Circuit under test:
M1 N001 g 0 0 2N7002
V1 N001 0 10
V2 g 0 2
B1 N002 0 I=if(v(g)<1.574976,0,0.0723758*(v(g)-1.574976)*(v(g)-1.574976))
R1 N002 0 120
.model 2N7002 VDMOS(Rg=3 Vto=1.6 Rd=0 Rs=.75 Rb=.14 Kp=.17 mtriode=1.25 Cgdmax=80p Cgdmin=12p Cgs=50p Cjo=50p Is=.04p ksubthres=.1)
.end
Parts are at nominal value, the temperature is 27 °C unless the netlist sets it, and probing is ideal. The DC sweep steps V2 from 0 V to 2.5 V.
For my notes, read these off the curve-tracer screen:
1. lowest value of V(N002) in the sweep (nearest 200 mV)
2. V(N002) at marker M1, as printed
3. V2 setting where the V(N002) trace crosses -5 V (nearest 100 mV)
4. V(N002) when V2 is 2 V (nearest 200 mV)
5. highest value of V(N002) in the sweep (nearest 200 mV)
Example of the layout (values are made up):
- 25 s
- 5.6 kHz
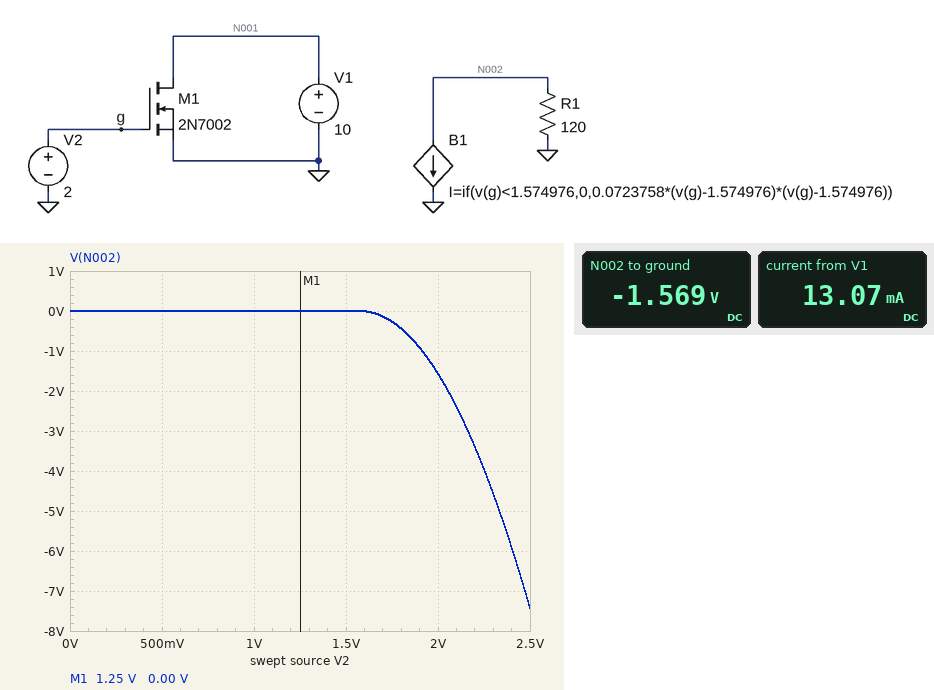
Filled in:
- -7.4 V
- 0.00 V
- 2.3 V
- -1.6 V
- 0 V
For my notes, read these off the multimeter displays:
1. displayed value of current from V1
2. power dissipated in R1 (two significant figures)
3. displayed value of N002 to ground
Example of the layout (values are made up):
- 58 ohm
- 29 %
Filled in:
- 13.07 mA
- 21 mW
- -1.569 V
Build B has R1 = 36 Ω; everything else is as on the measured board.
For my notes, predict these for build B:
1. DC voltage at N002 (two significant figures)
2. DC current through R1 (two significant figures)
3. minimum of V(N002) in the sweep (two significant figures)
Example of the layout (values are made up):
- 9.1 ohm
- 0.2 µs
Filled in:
- -470 mV
- 13 mA
- -2.2 V
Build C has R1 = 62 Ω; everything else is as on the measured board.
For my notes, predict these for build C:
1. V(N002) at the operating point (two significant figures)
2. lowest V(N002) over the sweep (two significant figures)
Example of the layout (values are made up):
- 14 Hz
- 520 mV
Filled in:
- -810 mV
- -3.8 V
